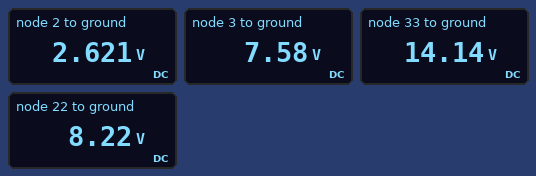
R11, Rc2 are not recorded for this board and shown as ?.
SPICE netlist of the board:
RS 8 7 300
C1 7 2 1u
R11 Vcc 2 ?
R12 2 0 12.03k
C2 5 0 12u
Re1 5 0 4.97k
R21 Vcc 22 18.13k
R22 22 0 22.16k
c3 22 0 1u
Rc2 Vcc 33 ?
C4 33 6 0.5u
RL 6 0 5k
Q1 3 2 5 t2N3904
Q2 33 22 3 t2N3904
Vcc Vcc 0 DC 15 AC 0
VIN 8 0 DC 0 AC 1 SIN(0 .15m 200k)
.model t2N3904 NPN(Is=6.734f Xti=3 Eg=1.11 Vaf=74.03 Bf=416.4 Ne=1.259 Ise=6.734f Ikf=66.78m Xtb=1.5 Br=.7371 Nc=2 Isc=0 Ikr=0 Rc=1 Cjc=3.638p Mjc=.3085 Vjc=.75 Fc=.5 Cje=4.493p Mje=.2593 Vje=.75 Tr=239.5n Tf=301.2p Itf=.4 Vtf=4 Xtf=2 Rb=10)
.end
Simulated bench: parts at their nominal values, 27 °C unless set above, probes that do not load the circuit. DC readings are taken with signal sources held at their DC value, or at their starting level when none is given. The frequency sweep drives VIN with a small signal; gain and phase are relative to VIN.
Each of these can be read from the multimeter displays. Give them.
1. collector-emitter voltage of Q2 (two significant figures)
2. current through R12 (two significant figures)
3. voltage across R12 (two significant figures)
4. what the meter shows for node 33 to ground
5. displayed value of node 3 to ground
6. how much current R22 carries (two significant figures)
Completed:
6.6 V
220 µA
2.6 V
14.14 V
7.58 V
370 µA
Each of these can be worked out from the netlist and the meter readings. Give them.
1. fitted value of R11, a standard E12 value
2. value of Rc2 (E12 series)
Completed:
56 kΩ
2.2 kΩ
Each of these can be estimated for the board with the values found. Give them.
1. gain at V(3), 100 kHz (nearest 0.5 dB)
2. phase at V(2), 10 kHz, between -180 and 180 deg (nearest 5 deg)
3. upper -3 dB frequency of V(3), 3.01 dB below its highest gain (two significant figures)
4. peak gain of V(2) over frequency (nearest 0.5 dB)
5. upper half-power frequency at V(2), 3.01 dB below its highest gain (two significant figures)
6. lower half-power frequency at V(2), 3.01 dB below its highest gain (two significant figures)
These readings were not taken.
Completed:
-0.5 dB
0 deg
38 MHz
-0.5 dB
36 MHz
16 Hz
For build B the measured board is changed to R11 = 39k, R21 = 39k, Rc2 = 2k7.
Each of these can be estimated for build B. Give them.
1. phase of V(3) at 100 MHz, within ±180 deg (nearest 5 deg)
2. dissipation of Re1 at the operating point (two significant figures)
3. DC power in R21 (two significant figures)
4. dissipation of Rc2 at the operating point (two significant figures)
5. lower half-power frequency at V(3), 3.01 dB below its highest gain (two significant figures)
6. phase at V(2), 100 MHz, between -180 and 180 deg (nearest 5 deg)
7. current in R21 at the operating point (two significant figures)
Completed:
90 deg
1.6 mW
2.4 mW
860 µW
300 Hz
-65 deg
250 µA
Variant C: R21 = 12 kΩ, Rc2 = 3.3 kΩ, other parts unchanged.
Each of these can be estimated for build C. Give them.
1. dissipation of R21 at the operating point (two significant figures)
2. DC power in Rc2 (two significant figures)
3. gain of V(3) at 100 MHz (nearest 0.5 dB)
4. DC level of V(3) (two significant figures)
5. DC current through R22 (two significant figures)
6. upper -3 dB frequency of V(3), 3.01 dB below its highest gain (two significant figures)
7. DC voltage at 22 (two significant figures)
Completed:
2.3 mW
510 µW
-9.5 dB
9.1 V
440 µA
40 MHz
9.7 V
